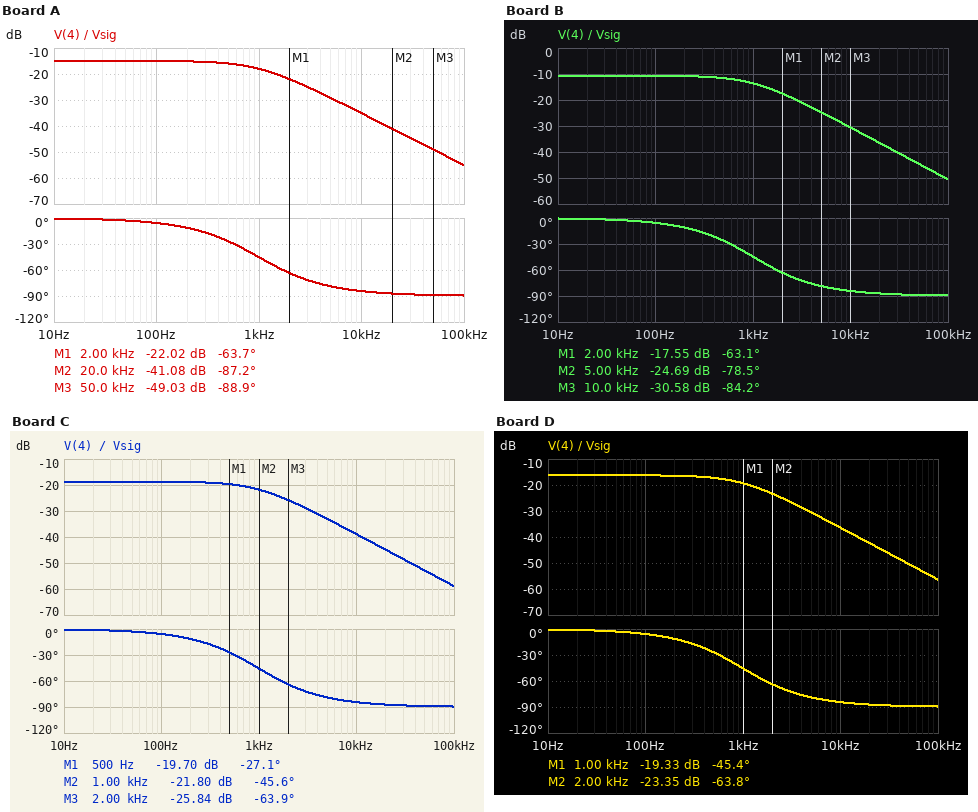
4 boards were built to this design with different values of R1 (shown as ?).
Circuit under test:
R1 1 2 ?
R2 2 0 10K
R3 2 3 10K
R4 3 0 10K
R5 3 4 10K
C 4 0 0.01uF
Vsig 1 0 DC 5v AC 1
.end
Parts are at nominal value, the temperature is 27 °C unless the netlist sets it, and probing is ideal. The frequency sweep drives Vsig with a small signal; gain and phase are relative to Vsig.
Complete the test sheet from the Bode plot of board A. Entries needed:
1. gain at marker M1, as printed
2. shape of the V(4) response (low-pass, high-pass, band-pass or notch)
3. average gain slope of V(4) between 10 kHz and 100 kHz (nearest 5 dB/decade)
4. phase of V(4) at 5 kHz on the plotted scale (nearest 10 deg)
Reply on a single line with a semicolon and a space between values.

-22.02 dB; low-pass; -20 dB/decade; -80 deg
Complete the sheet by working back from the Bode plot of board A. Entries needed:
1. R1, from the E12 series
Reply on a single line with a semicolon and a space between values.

12 kΩ
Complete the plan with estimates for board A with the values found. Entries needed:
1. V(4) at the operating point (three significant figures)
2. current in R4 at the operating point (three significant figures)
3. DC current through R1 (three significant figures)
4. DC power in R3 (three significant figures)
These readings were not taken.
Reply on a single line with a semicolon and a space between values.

893 mV; 89.3 µA; 268 µA; 79.7 µW
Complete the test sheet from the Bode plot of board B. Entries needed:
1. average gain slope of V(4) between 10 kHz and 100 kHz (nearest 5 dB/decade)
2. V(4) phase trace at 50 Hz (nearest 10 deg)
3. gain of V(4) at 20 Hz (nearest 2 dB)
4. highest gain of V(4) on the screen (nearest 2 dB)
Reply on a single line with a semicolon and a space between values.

-20 dB/decade; 0 deg; -10 dB; -10 dB
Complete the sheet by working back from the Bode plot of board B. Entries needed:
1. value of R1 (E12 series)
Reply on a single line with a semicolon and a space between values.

4.7 kΩ
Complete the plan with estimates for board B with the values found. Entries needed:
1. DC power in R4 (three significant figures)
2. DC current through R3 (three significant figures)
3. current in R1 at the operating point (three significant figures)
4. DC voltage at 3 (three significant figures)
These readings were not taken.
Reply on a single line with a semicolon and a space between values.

215 µW; 147 µA; 440 µA; 1.47 V
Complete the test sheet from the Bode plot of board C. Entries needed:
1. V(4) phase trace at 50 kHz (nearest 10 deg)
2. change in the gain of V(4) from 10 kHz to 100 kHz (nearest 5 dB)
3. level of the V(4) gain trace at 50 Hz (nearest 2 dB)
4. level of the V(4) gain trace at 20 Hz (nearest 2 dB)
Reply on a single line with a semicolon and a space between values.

-90 deg; -20 dB; -18 dB; -18 dB
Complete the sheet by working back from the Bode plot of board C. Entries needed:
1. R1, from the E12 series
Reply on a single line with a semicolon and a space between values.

22 kΩ
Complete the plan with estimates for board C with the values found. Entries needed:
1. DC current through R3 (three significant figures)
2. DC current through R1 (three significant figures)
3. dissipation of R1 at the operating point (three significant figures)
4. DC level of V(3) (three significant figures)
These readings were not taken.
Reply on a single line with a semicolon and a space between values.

58.1 µA; 174 µA; 669 µW; 581 mV
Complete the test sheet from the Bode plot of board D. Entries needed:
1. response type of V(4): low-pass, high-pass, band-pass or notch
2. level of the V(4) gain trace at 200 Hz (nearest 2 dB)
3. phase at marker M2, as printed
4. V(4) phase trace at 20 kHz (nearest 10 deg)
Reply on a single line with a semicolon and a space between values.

low-pass; -16 dB; -63.8 deg; -90 deg
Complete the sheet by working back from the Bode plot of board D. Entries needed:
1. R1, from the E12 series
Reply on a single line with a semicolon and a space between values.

15 kΩ
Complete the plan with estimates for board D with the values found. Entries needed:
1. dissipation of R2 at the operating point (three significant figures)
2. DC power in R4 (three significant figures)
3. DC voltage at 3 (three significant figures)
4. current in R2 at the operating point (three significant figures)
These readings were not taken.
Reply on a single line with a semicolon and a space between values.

237 µW; 59.2 µW; 769 mV; 154 µA
